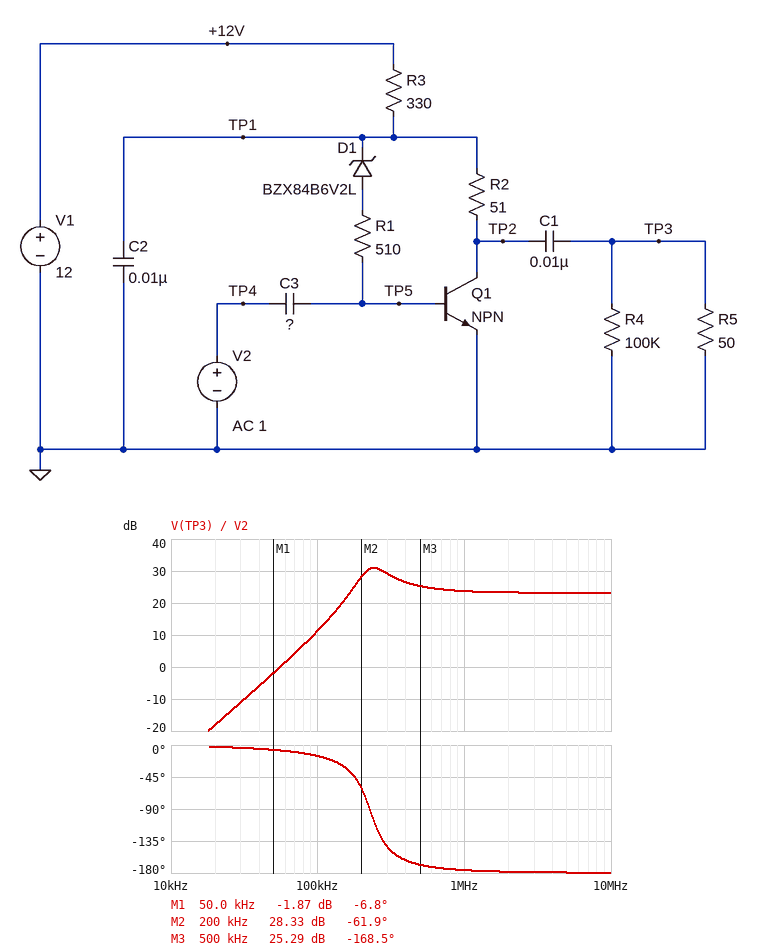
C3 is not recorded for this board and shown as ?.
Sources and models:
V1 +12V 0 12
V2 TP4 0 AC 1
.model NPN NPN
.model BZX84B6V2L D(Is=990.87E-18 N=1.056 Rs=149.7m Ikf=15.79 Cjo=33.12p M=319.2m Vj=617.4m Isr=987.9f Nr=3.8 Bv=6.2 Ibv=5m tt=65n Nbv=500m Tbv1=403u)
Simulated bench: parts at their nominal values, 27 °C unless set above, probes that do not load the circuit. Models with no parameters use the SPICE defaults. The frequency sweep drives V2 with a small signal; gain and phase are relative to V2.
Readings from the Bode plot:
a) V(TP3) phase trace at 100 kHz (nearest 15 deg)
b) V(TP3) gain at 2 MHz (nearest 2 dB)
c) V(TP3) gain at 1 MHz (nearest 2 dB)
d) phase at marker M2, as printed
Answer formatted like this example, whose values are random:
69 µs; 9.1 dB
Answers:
-15 deg; 24 dB; 24 dB; -61.9 deg
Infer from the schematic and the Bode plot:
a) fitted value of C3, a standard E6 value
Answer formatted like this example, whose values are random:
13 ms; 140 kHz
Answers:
22 nF
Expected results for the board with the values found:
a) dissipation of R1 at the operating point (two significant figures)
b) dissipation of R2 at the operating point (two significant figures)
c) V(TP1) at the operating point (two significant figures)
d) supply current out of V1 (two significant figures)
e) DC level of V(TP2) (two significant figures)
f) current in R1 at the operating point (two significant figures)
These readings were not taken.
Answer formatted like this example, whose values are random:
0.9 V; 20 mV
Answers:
11 µW; 11 mW; 7.1 V; 15 mA; 6.3 V; 150 µA
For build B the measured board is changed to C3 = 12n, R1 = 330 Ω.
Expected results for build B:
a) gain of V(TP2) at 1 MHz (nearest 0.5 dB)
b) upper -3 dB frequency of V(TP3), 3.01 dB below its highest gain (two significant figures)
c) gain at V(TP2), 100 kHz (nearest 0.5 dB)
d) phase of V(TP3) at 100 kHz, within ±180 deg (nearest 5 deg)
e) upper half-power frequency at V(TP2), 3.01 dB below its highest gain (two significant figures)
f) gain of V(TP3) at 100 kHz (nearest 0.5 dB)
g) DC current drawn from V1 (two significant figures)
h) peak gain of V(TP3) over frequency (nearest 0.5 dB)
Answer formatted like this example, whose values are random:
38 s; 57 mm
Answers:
25.0 dB; 580 kHz; 12.5 dB; -10 deg; 530 kHz; 2.0 dB; 15 mA; 30.0 dB
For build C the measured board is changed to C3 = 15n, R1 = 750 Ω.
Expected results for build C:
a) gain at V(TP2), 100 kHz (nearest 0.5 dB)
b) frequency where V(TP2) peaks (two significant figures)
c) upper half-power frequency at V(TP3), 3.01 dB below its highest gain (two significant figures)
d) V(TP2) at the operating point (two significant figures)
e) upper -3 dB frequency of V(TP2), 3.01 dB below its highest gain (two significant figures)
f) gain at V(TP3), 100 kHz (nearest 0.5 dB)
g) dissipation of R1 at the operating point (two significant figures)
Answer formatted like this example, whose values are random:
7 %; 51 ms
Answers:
21.0 dB; 240 kHz; 370 kHz; 6.4 V; 320 kHz; 10.5 dB; 16 µW
